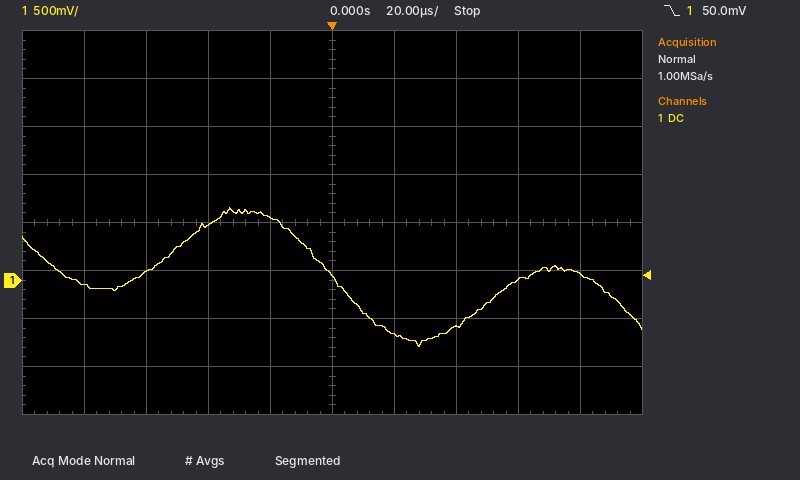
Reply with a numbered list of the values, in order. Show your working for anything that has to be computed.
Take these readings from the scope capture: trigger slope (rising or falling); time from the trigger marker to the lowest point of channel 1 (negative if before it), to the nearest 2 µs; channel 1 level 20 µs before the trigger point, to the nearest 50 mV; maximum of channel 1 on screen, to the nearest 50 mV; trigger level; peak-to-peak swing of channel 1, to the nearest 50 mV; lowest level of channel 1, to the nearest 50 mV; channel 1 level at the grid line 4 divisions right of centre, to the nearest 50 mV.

1. falling
2. +28 µs
3. 650 mV
4. 750 mV
5. 50.0 mV
6. 750 mV − (-700 mV) = 1.45 V
7. -700 mV
8. 50 mV
